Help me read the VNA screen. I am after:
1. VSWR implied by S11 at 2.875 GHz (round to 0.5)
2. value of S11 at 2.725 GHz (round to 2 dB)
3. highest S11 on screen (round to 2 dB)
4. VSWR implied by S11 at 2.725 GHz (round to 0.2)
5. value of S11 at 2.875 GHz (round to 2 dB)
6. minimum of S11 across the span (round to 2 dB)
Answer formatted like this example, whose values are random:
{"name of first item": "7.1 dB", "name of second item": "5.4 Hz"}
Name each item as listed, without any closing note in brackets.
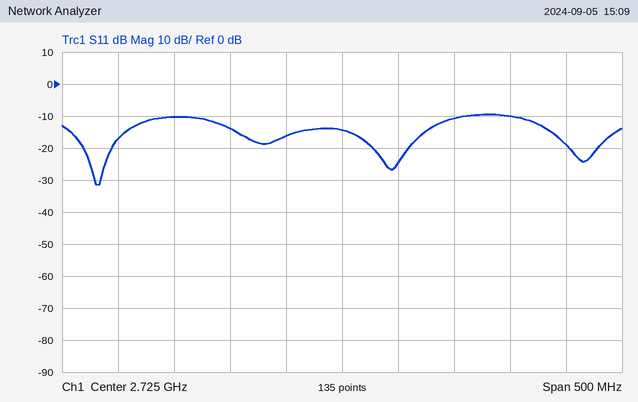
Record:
{"VSWR implied by S11 at 2.875 GHz": "2.0", "value of S11 at 2.725 GHz": "-14 dB", "highest S11 on screen": "-10 dB", "VSWR implied by S11 at 2.725 GHz": "1.4", "value of S11 at 2.875 GHz": "-10 dB", "minimum of S11 across the span": "-32 dB"}
